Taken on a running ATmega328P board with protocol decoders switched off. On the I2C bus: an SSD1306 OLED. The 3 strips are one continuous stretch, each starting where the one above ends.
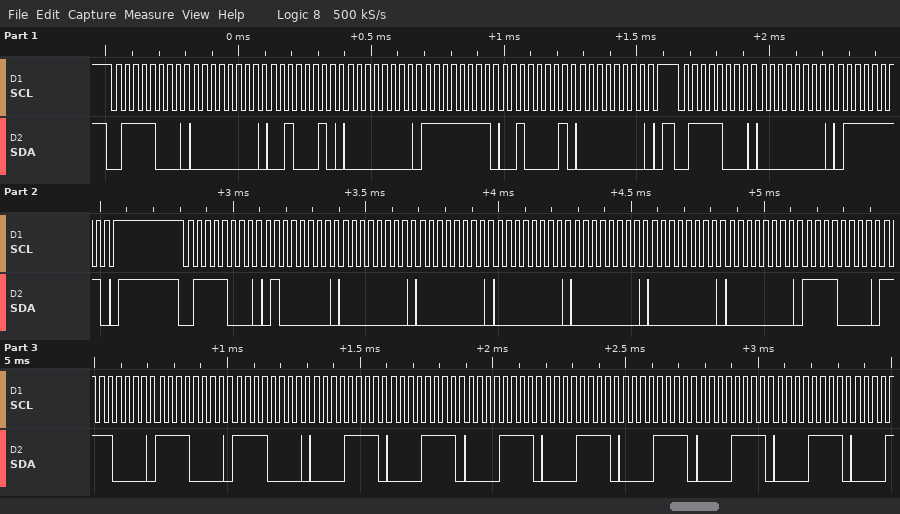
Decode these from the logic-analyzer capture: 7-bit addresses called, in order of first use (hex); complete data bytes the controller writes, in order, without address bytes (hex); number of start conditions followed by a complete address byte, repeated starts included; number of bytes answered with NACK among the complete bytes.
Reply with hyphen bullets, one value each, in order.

- 0x3C
- 00 22 00 FF 21 00 00 7F 40 00 00 00 00 00 00 F0 F0 F0 F0 0F 0F 0F 0F 0F 0F 0F
- 3
- 0
